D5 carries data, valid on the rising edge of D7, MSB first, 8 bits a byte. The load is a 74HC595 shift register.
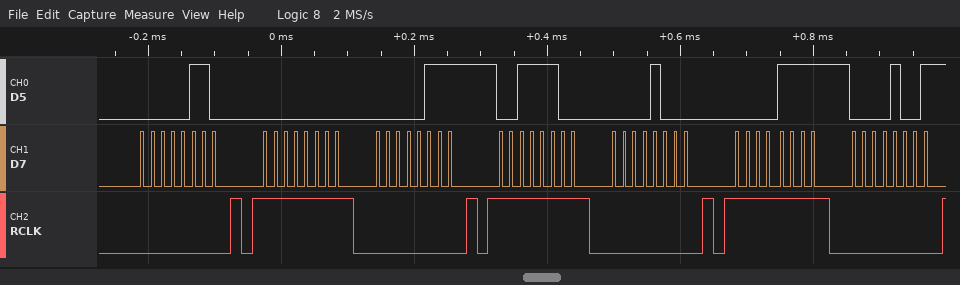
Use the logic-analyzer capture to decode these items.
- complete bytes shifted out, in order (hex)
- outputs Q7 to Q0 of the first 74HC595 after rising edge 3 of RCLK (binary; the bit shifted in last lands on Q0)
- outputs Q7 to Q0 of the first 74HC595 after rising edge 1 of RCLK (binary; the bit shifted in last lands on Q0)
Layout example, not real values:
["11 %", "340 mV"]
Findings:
["06 00 07 3C 08 0F 09", "00000111", "00000110"]
